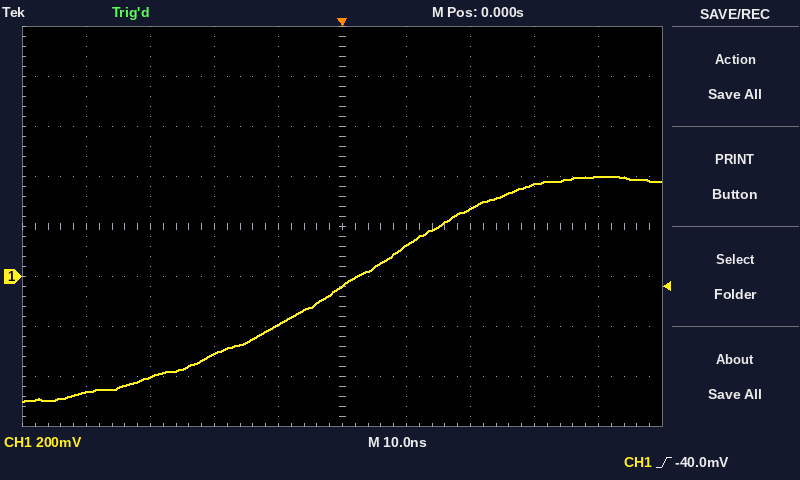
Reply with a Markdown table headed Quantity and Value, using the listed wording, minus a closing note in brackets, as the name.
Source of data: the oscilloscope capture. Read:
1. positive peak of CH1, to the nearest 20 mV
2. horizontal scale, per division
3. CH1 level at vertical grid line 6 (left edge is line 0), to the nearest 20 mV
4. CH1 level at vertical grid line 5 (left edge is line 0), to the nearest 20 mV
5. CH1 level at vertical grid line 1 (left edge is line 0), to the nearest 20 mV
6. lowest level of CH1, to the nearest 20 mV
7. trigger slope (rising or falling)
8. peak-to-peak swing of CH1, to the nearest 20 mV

| Quantity | Value |
|---|---|
| positive peak of CH1, to the nearest 20 mV | 400 mV |
| horizontal scale, per division | 10 ns |
| CH1 level at vertical grid line 6 (left edge is line 0), to the nearest 20 mV | 120 mV |
| CH1 level at vertical grid line 5 (left edge is line 0), to the nearest 20 mV | -40 mV |
| CH1 level at vertical grid line 1 (left edge is line 0), to the nearest 20 mV | -460 mV |
| lowest level of CH1, to the nearest 20 mV | -500 mV |
| trigger slope | rising |
| peak-to-peak swing of CH1, to the nearest 20 mV | 900 mV |
